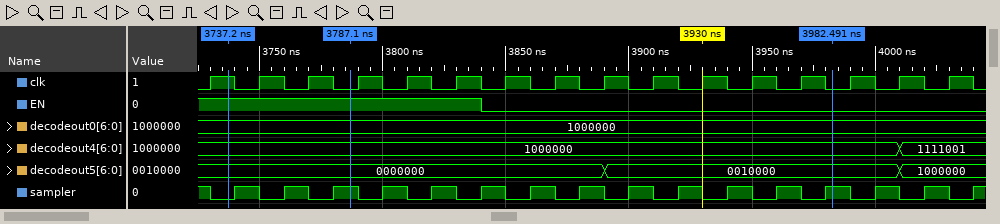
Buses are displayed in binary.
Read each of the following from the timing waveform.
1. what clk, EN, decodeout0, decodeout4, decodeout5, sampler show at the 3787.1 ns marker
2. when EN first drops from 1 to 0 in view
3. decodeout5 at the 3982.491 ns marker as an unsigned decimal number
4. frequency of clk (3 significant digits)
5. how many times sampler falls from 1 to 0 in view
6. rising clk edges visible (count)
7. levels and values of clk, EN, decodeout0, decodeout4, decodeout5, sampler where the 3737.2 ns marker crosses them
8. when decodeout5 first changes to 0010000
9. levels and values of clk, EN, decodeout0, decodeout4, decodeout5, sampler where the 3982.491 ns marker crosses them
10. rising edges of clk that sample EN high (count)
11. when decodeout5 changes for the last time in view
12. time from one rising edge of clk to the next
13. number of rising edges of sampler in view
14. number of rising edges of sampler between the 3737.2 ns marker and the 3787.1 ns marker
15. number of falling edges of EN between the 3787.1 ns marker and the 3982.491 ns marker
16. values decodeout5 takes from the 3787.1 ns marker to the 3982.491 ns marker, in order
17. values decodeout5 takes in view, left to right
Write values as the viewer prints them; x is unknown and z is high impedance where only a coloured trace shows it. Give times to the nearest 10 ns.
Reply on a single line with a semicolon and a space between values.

clk=0, EN=1, decodeout0=1000000, decodeout4=1000000, decodeout5=0000000, sampler=1; 3840 ns; 16; 50.0 MHz; 16; 16; clk=1, EN=1, decodeout0=1000000, decodeout4=1000000, decodeout5=0000000, sampler=0; 3890 ns; clk=0, EN=0, decodeout0=1000000, decodeout4=1000000, decodeout5=0010000, sampler=1; 6; 4010 ns; 20 ns; 16; 3; 1; 0000000, 0010000; 0000000, 0010000, 1000000
